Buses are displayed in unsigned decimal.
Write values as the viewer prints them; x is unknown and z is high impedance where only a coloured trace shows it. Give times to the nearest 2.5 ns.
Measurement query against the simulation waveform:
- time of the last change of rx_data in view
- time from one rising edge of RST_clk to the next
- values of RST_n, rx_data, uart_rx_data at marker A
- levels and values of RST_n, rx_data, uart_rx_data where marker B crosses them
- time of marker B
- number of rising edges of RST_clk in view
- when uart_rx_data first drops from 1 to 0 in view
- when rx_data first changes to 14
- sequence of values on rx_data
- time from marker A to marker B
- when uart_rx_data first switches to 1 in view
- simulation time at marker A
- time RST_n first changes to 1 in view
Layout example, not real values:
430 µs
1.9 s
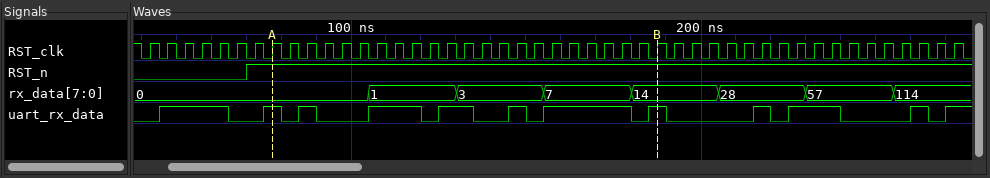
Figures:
255 ns
5 ns
RST_n=1, rx_data=0, uart_rx_data=1
RST_n=1, rx_data=14, uart_rx_data=1
187.5 ns
47
65 ns
180 ns
0, 1, 3, 7, 14, 28, 57, 114
110 ns
45 ns
77.5 ns
70 ns
